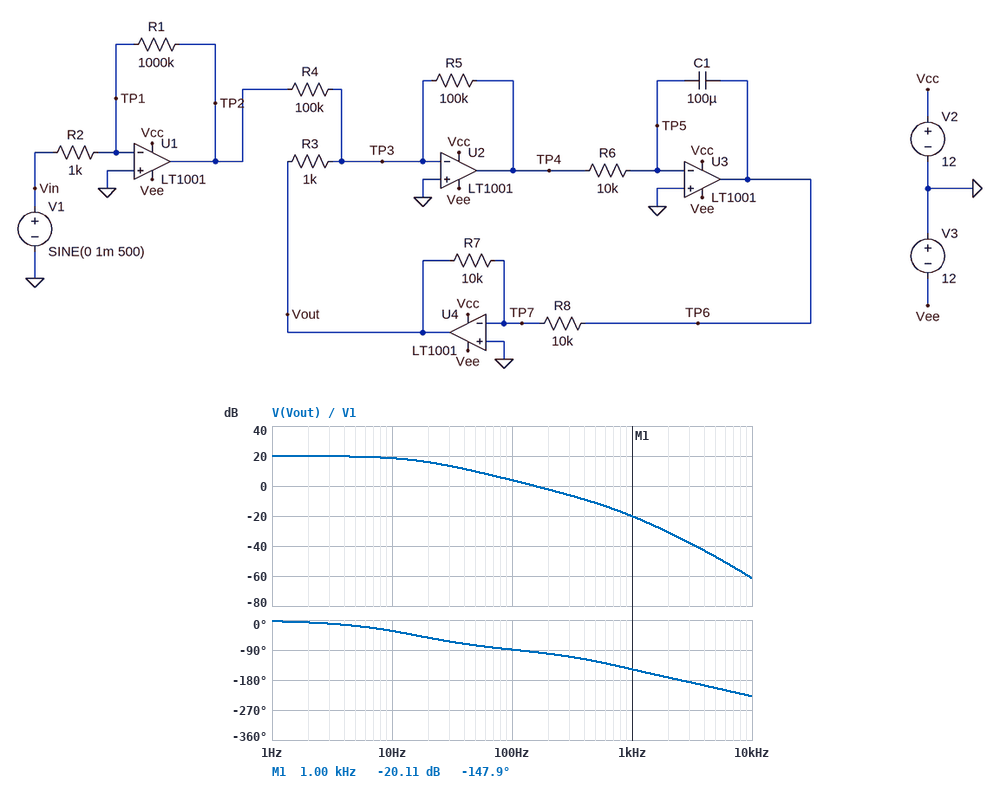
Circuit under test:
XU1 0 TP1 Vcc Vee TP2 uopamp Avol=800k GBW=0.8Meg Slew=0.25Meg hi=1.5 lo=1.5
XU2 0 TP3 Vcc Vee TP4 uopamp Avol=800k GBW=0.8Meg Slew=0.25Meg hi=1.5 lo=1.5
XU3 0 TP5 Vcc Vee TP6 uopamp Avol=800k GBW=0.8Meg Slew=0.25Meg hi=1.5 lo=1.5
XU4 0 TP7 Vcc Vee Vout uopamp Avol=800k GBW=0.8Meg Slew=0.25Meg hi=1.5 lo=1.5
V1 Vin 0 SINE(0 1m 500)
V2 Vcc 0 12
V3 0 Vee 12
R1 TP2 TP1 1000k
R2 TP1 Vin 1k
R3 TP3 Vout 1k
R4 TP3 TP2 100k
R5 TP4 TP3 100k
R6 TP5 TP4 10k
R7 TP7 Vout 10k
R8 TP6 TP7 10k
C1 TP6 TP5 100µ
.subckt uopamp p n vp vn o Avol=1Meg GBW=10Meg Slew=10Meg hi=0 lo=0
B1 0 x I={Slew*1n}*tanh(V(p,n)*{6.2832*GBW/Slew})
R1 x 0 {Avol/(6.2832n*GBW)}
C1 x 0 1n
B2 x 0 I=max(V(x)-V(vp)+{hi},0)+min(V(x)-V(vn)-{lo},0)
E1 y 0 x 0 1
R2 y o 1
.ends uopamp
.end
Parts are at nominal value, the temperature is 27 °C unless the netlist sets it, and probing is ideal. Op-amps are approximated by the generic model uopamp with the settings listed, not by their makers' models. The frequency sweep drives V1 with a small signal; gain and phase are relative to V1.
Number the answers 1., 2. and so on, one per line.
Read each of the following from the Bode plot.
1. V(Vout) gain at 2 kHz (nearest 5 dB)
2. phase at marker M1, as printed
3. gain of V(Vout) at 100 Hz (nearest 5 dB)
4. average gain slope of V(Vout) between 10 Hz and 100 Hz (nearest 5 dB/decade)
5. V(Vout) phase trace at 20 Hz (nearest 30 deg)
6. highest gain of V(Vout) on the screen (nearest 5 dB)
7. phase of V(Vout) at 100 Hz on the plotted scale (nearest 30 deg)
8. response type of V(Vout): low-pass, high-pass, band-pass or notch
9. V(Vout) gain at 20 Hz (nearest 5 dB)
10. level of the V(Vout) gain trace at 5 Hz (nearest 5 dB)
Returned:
1. -30 dB
2. -147.9 deg
3. 5 dB
4. -15 dB/decade
5. -60 deg
6. 20 dB
7. -90 deg
8. low-pass
9. 15 dB
10. 20 dB
